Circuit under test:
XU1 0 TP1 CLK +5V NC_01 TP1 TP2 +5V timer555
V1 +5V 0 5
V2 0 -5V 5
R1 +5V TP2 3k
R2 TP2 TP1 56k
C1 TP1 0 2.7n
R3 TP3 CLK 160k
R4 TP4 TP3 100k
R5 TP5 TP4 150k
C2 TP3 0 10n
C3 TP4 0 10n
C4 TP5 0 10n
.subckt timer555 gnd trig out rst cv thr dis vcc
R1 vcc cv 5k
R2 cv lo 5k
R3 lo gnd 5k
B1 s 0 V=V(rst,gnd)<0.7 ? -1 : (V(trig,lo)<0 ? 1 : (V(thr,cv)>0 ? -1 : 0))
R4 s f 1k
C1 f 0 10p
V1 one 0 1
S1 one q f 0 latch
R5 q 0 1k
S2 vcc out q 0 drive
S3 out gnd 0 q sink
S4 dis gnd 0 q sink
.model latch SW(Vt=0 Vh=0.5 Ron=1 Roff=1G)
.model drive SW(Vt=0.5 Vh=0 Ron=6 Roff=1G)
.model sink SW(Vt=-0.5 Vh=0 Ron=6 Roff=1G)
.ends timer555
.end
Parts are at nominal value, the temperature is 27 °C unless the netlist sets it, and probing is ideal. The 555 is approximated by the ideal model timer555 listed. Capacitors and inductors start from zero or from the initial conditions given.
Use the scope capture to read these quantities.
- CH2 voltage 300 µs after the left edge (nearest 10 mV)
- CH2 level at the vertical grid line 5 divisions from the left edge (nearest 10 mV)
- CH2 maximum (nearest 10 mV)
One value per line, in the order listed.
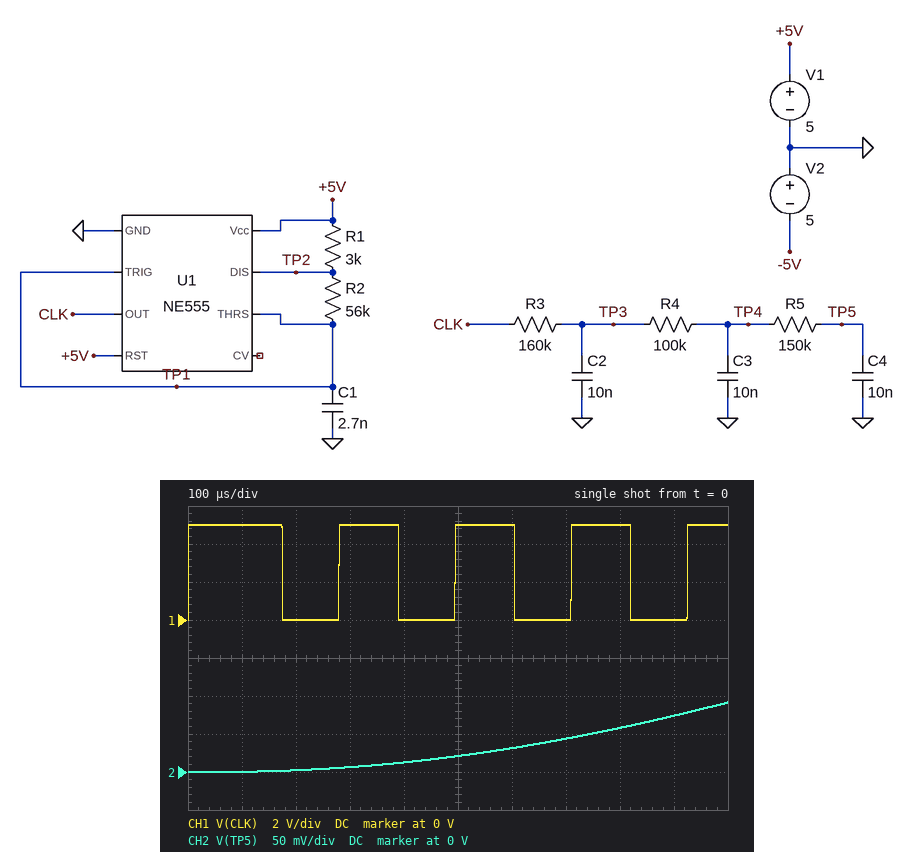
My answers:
10 mV
20 mV
90 mV
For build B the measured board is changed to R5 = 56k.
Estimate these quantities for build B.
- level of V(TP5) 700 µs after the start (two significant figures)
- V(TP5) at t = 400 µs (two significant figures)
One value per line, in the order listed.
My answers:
84 mV
27 mV
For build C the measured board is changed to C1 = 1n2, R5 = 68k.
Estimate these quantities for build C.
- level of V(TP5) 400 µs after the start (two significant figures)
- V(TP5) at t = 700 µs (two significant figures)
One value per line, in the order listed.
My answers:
19 mV
65 mV
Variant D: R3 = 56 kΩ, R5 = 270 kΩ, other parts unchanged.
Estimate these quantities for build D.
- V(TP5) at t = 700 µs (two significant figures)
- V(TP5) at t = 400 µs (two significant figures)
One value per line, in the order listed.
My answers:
64 mV
19 mV
